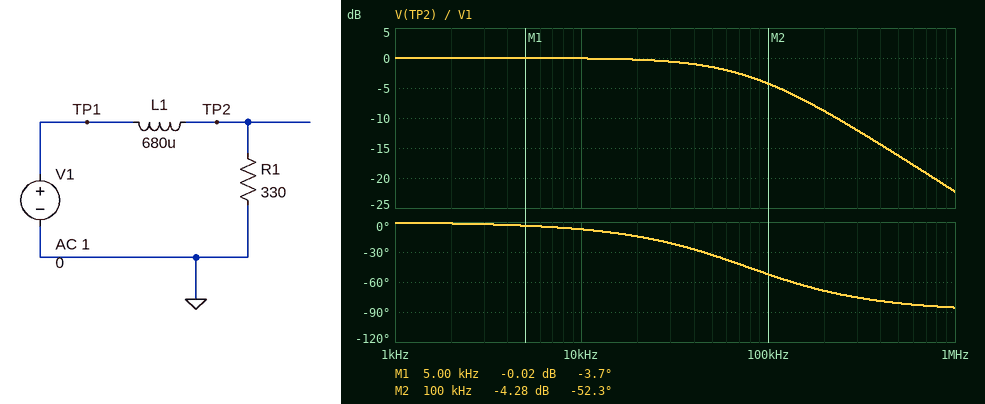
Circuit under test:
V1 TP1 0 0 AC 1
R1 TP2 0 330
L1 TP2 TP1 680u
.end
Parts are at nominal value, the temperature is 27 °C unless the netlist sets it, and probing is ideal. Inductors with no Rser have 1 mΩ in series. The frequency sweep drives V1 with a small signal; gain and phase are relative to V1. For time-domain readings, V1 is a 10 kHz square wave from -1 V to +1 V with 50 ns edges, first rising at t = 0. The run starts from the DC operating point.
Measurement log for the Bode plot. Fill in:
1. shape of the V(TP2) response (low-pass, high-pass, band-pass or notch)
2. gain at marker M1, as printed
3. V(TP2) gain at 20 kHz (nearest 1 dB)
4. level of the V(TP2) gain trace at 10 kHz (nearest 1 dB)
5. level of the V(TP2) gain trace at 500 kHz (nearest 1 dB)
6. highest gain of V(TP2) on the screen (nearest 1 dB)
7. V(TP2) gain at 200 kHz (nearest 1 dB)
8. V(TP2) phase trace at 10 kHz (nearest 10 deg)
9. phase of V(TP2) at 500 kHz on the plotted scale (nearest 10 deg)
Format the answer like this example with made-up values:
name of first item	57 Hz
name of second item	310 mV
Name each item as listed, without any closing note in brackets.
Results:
shape of the V(TP2) response	low-pass
gain at marker M1, as printed	-0.02 dB
V(TP2) gain at 20 kHz	0 dB
level of the V(TP2) gain trace at 10 kHz	0 dB
level of the V(TP2) gain trace at 500 kHz	-16 dB
highest gain of V(TP2) on the screen	0 dB
V(TP2) gain at 200 kHz	-9 dB
V(TP2) phase trace at 10 kHz	-10 deg
phase of V(TP2) at 500 kHz on the plotted scale	-80 deg
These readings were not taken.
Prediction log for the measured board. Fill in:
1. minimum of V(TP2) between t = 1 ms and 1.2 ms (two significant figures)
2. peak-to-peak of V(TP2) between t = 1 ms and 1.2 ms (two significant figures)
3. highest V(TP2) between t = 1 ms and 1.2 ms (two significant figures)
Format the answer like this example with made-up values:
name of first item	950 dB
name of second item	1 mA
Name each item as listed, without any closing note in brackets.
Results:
minimum of V(TP2) between t = 1 ms and 1.2 ms	-1.0 V
peak-to-peak of V(TP2) between t = 1 ms and 1.2 ms	2.0 V
highest V(TP2) between t = 1 ms and 1.2 ms	1.0 V
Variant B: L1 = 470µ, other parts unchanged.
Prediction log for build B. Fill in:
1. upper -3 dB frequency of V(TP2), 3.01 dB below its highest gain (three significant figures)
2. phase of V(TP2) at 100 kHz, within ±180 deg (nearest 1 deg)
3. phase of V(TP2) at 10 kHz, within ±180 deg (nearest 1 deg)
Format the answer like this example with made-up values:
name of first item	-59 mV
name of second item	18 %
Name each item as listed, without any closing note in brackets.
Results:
upper -3 dB frequency of V(TP2), 3.01 dB below its highest gain	112 kHz
phase of V(TP2) at 100 kHz, within ±180 deg	-42 deg
phase of V(TP2) at 10 kHz, within ±180 deg	-5 deg
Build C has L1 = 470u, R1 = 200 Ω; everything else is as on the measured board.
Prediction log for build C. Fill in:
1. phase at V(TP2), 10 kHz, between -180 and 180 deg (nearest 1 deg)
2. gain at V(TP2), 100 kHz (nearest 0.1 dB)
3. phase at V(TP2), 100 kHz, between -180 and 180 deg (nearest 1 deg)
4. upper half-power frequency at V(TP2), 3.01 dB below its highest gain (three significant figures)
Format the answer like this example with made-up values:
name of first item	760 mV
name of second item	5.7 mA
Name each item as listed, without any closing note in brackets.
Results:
phase at V(TP2), 10 kHz, between -180 and 180 deg	-8 deg
gain at V(TP2), 100 kHz	-5.0 dB
phase at V(TP2), 100 kHz, between -180 and 180 deg	-56 deg
upper half-power frequency at V(TP2), 3.01 dB below its highest gain	67.7 kHz
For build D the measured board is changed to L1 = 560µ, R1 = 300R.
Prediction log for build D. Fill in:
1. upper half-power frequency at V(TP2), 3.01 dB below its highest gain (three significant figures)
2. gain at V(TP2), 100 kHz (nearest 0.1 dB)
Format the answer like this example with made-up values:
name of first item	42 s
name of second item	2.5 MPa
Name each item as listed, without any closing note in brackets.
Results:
upper half-power frequency at V(TP2), 3.01 dB below its highest gain	85.3 kHz
gain at V(TP2), 100 kHz	-3.8 dB
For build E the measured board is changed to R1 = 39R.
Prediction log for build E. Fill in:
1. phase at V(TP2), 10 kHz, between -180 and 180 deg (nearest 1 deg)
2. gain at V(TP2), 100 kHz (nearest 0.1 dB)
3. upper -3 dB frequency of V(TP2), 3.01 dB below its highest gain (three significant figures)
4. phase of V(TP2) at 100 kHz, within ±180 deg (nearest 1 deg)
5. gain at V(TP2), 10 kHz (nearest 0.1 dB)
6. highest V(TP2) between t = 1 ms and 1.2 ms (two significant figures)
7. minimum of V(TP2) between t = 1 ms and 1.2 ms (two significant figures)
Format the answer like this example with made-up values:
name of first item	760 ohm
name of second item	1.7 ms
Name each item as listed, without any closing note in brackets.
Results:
phase at V(TP2), 10 kHz, between -180 and 180 deg	-48 deg
gain at V(TP2), 100 kHz	-20.8 dB
upper -3 dB frequency of V(TP2), 3.01 dB below its highest gain	9.13 kHz
phase of V(TP2) at 100 kHz, within ±180 deg	-85 deg
gain at V(TP2), 10 kHz	-3.4 dB
highest V(TP2) between t = 1 ms and 1.2 ms	890 mV
minimum of V(TP2) between t = 1 ms and 1.2 ms	-890 mV
